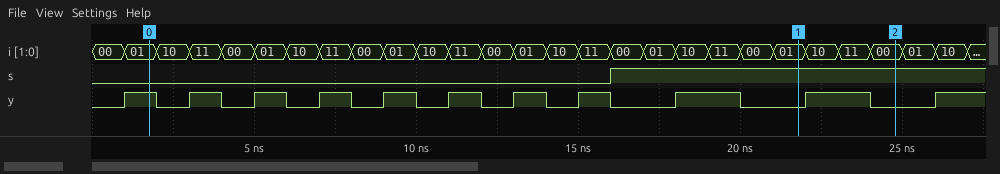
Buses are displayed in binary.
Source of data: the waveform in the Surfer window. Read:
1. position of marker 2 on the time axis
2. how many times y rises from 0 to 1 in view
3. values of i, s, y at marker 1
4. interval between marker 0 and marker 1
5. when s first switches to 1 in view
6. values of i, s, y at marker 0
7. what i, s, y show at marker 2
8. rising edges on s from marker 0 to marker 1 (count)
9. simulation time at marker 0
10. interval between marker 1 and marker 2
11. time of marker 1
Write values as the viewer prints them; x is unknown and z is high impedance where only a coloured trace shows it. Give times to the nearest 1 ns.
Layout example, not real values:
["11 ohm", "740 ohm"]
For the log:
["25 ns", "11", "i=01, s=1, y=0", "20 ns", "16 ns", "i=01, s=0, y=1", "i=00, s=1, y=0", "1", "2 ns", "3 ns", "22 ns"]
